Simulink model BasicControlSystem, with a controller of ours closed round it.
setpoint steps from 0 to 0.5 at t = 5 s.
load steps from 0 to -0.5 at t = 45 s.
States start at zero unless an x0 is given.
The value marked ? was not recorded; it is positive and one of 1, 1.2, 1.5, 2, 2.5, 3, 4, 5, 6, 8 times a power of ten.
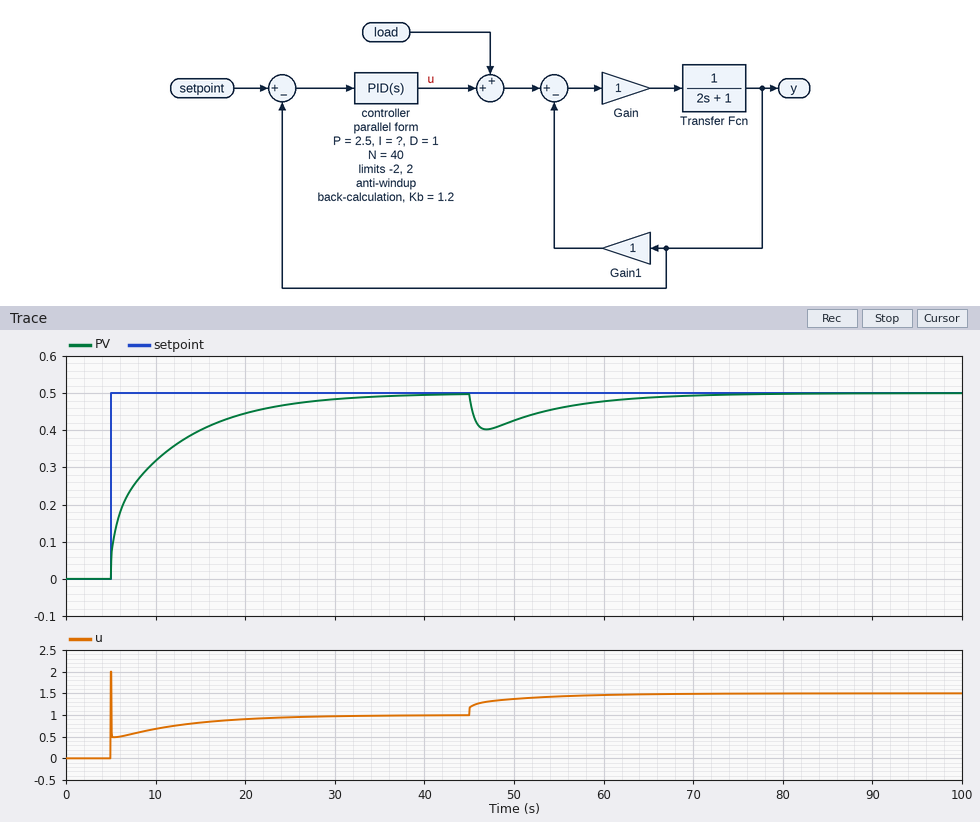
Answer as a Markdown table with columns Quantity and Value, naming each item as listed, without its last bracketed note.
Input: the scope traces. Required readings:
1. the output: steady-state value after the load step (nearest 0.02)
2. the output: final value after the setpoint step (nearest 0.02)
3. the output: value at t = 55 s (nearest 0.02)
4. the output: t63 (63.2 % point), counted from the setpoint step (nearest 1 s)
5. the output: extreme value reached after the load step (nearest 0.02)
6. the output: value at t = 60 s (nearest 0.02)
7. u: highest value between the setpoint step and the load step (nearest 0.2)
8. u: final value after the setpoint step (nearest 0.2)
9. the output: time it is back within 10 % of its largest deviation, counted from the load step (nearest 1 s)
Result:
| Quantity | Value |
|---|---|
| the output: steady-state value after the load step | 0.50 |
| the output: final value after the setpoint step | 0.50 |
| the output: value at t = 55 s | 0.46 |
| the output: t63 (63.2 % point), counted from the setpoint step | 5 s |
| the output: extreme value reached after the load step | 0.40 |
| the output: value at t = 60 s | 0.48 |
| u: highest value between the setpoint step and the load step | 2.0 |
| u: final value after the setpoint step | 1.0 |
| the output: time it is back within 10 % of its largest deviation, counted from the load step | 22 s |
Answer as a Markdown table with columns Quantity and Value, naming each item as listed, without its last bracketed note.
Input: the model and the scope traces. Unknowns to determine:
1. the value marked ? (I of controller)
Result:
| Quantity | Value |
|---|---|
| the value marked ? | 0.5 |
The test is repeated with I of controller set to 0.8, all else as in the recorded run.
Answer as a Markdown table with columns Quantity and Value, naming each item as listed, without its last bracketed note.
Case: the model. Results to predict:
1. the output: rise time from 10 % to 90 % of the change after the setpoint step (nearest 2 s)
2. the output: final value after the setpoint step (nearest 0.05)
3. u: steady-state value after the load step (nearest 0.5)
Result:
| Quantity | Value |
|---|---|
| the output: rise time from 10 % to 90 % of the change after the setpoint step | 10 s |
| the output: final value after the setpoint step | 0.50 |
| u: steady-state value after the load step | 1.5 |
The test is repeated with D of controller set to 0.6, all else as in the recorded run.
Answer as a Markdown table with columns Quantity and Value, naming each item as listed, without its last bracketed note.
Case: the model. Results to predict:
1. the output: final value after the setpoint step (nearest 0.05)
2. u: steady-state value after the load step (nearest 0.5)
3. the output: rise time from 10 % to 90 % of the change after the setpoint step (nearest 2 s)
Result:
| Quantity | Value |
|---|---|
| the output: final value after the setpoint step | 0.50 |
| u: steady-state value after the load step | 1.5 |
| the output: rise time from 10 % to 90 % of the change after the setpoint step | 14 s |
